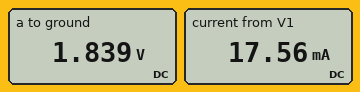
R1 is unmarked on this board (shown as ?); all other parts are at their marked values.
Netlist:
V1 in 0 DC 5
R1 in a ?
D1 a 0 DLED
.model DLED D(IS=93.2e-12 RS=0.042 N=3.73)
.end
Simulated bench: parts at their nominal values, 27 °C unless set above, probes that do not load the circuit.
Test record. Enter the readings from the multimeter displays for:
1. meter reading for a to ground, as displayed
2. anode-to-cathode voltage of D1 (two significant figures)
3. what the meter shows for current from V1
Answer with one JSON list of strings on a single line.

["1.839 V", "1.8 V", "17.56 mA"]
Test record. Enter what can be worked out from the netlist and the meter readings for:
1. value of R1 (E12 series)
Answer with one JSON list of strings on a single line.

["180 Ω"]
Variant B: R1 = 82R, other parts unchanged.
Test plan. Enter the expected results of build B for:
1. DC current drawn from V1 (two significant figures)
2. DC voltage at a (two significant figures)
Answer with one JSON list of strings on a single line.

["38 mA", "1.9 V"]
